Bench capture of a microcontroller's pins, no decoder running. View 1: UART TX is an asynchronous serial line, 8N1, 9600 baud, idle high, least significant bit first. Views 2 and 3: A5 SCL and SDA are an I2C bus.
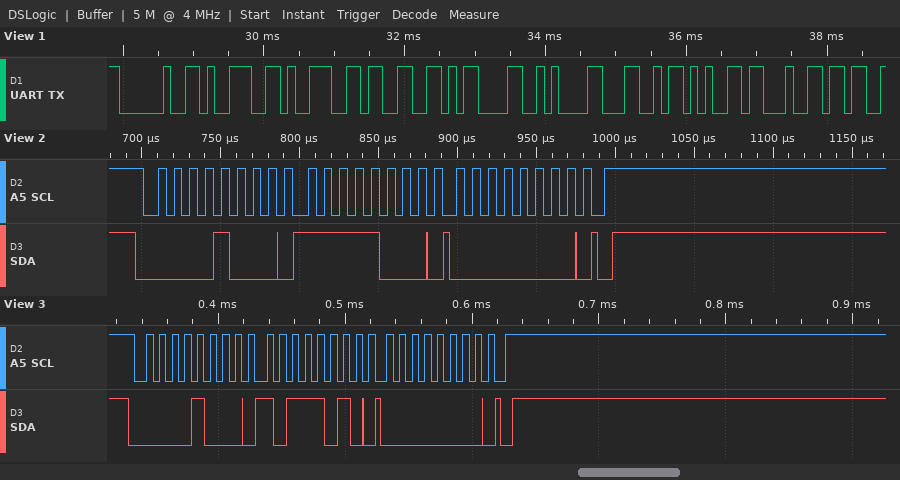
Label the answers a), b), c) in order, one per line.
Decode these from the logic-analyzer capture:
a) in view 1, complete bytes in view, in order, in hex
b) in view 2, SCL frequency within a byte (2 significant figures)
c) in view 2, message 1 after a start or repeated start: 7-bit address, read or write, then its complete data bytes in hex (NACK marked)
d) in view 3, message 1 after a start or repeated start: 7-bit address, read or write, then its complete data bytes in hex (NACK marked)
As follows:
a) 20 39 39 33 0D 0A 4C 65 64
b) 100 kHz
c) 0x04 write: F8 00
d) 0x04 write: BA 00
